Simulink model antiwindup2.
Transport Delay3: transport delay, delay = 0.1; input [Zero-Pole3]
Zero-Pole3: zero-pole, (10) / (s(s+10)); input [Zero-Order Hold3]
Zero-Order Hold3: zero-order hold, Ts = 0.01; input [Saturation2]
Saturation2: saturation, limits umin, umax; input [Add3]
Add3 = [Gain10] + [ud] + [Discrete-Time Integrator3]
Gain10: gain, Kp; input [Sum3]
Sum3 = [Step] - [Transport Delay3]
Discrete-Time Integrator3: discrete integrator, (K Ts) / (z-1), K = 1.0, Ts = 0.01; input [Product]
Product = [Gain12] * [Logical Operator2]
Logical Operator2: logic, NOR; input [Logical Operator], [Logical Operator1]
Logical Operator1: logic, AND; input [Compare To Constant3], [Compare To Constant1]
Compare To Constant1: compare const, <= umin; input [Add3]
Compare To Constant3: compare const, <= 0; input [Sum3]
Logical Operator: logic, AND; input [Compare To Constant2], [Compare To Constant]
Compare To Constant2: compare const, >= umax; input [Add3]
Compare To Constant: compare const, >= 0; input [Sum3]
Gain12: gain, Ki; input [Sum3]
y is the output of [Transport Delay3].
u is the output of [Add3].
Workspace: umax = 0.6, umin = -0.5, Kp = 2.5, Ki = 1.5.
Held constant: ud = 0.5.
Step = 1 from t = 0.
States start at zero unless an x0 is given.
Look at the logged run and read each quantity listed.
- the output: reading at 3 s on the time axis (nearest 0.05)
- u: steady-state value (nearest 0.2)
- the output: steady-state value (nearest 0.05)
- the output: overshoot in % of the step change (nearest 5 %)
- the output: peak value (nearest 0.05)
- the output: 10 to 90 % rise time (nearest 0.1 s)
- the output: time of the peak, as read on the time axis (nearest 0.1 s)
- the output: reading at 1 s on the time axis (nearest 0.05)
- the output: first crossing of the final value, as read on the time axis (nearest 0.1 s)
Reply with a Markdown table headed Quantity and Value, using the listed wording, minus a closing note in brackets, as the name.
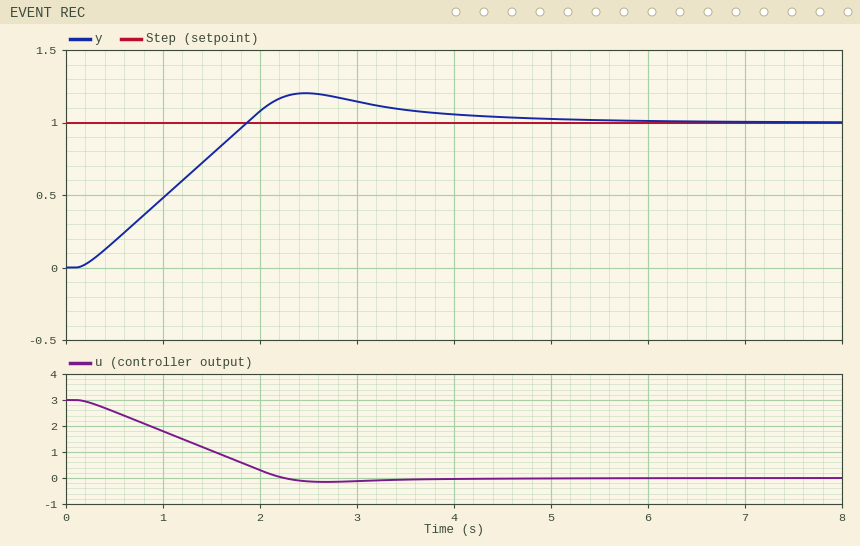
| Quantity | Value |
|---|---|
| the output: reading at 3 s on the time axis | 1.15 |
| u: steady-state value | 0.0 |
| the output: steady-state value | 1.00 |
| the output: overshoot in % of the step change | 20 % |
| the output: peak value | 1.20 |
| the output: 10 to 90 % rise time | 1.3 s |
| the output: time of the peak, as read on the time axis | 2.5 s |
| the output: reading at 1 s on the time axis | 0.50 |
| the output: first crossing of the final value, as read on the time axis | 1.9 s |
